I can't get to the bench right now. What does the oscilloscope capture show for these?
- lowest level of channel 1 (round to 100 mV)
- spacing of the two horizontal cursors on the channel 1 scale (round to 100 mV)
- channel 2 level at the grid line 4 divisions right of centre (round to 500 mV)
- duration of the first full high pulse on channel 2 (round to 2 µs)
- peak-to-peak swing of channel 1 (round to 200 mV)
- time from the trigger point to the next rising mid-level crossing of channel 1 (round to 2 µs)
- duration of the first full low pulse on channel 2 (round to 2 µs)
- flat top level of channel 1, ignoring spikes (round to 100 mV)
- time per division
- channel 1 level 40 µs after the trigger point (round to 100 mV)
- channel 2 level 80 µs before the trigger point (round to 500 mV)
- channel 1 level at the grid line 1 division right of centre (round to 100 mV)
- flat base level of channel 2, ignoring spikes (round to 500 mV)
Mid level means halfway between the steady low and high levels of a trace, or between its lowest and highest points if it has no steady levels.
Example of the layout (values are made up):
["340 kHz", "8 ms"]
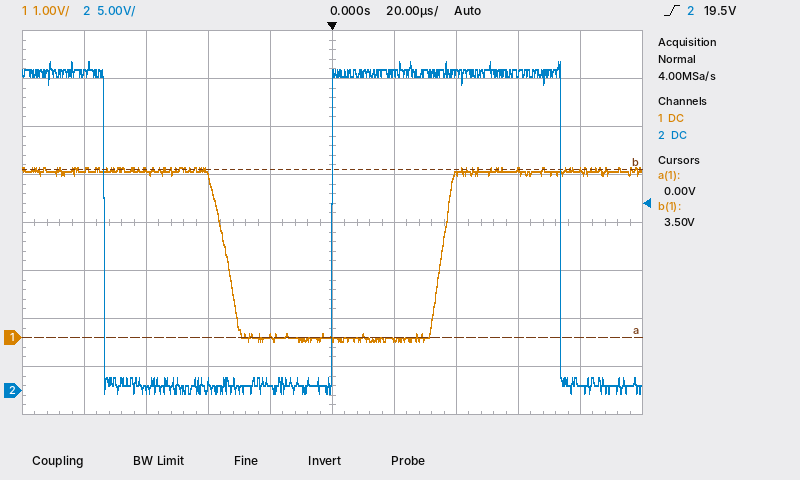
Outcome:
["-100 mV", "3.5 V", "500 mV", "74 µs", "3.6 V", "36 µs", "74 µs", "3.5 V", "20 µs", "3.4 V", "33.0 V", "0.0 V", "500 mV"]
